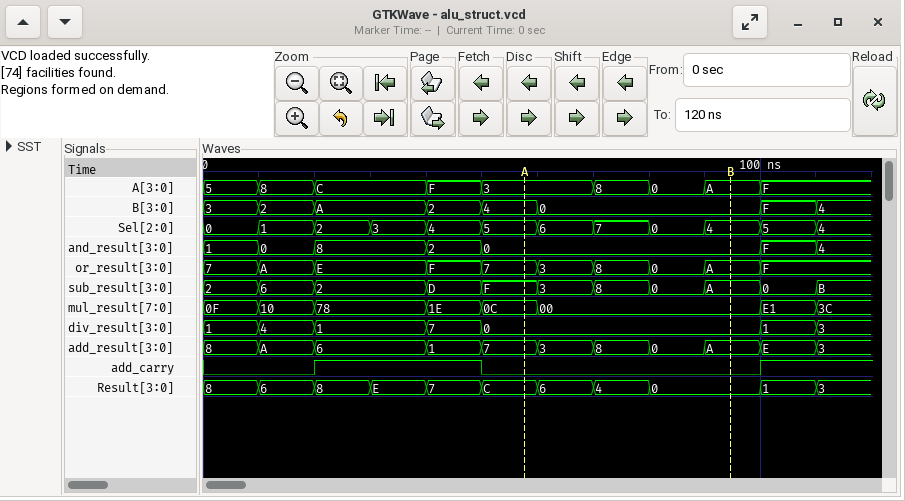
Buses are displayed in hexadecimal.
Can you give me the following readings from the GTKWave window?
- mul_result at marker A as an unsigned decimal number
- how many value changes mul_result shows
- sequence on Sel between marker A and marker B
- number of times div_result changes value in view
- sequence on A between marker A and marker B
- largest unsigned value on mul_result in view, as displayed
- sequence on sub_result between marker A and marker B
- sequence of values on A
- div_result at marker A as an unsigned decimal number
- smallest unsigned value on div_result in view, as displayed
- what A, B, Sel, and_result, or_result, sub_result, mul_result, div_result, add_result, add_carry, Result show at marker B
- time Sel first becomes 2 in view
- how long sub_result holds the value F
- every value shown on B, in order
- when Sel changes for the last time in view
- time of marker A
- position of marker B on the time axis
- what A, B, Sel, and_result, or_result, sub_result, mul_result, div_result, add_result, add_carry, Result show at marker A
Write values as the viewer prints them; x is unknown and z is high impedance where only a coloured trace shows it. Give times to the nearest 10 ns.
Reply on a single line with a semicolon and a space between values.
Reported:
12; 7; 5, 6, 7, 0, 4; 6; 3, 8, 0, A; E1; F, 3, 8, 0, A; 5, 8, C, F, 3, 8, 0, A, F; 0; 0; A=A, B=0, Sel=4, and_result=0, or_result=A, sub_result=A, mul_result=00, div_result=0, add_result=A, add_carry=0, Result=0; 20 ns; 10 ns; 3, 2, A, 2, 4, 0, F, 4; 110 ns; 60 ns; 90 ns; A=3, B=4, Sel=5, and_result=0, or_result=7, sub_result=F, mul_result=0C, div_result=0, add_result=7, add_carry=0, Result=C
